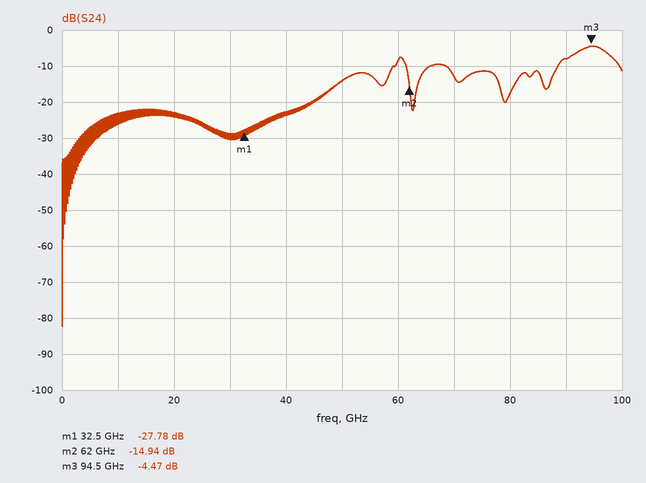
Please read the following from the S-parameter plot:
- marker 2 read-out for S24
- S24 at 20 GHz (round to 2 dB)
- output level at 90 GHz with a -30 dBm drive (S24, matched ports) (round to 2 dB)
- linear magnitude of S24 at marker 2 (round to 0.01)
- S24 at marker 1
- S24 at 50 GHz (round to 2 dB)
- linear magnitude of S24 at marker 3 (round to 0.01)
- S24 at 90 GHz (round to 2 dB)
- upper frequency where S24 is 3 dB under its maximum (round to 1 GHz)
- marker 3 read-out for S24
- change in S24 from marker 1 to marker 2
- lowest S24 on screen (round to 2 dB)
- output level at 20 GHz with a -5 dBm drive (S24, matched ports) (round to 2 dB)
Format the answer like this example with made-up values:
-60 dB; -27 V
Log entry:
-14.94 dB; -24 dB; -38 dBm; 0.18; -27.78 dB; -14 dB; 0.60; -8 dB; 98 GHz; -4.47 dB; 12.84 dB; -82 dB; -28 dBm
